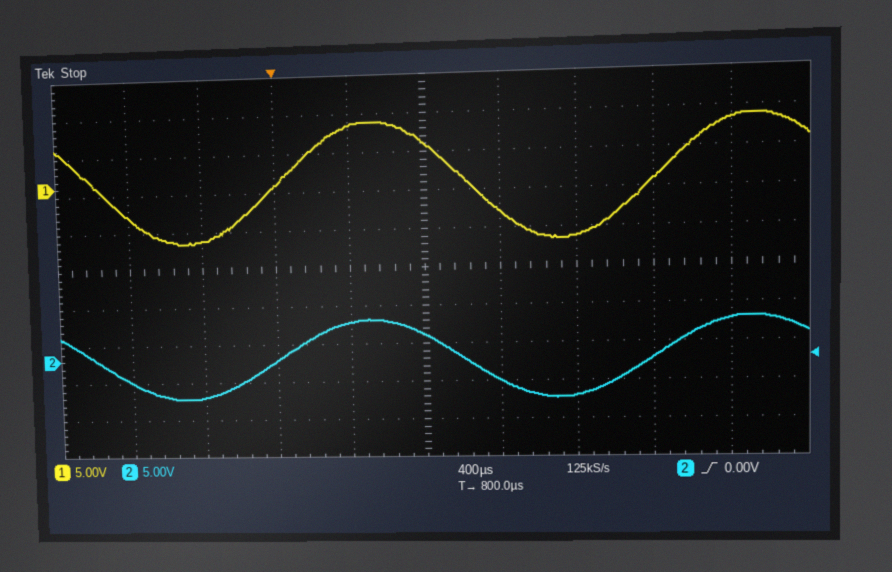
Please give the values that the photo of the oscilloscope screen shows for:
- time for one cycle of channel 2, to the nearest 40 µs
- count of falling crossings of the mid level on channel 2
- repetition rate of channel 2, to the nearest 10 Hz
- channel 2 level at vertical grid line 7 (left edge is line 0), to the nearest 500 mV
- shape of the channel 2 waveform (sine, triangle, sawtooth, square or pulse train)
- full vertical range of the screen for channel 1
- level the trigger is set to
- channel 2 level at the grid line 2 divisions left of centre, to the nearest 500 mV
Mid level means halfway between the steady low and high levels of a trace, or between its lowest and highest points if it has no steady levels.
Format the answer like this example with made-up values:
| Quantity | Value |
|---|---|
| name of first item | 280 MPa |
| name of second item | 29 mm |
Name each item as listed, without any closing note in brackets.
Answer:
| Quantity | Value |
|---|---|
| time for one cycle of channel 2, to the nearest 40 µs | 2.00 ms |
| count of falling crossings of the mid level on channel 2 | 2 |
| repetition rate of channel 2, to the nearest 10 Hz | 500 Hz |
| channel 2 level at vertical grid line 7 (left edge is line 0), to the nearest 500 mV | -5.0 V |
| shape of the channel 2 waveform | sine |
| full vertical range of the screen for channel 1 | 50 V |
| level the trigger is set to | 0.00 V |
| channel 2 level at the grid line 2 divisions left of centre, to the nearest 500 mV | 0.0 V |
